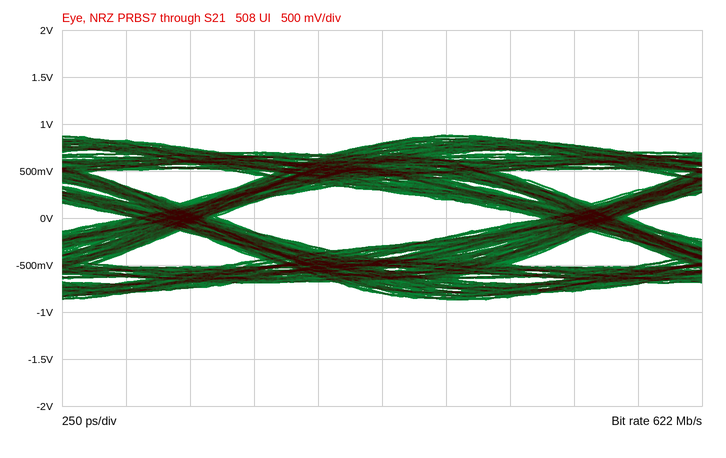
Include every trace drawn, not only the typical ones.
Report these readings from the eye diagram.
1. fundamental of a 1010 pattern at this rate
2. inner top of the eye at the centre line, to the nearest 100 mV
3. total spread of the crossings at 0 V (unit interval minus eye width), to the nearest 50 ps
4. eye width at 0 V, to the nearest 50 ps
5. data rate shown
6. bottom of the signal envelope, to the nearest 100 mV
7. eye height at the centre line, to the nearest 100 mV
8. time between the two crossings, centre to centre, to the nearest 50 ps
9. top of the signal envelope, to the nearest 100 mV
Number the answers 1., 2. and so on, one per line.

1. 311 MHz
2. 300 mV
3. 350 ps
4. 1.25 ns
5. 622 Mb/s
6. -900 mV
7. 600 mV
8. 1.60 ns
9. 900 mV
